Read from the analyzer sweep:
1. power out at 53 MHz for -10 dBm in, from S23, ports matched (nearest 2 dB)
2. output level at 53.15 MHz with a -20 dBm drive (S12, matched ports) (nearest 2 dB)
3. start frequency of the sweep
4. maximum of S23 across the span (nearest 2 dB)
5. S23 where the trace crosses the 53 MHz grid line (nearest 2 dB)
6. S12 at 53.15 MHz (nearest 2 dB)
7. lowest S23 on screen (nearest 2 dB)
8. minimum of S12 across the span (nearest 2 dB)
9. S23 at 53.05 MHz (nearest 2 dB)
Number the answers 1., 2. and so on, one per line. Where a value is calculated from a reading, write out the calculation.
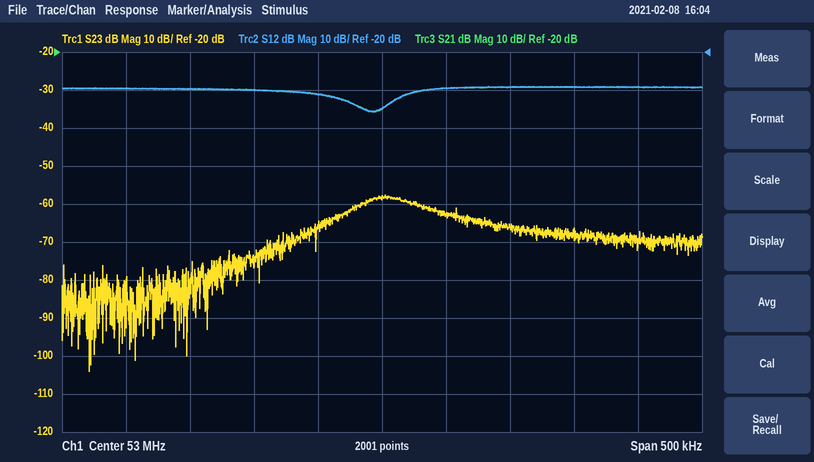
1. -10 dBm + (-58 dB) = -68 dBm
2. -20 dBm + (-30 dB) = -50 dBm
3. 52.75 MHz
4. -58 dB
5. -58 dB
6. -30 dB
7. -104 dB
8. -36 dB
9. -62 dB
